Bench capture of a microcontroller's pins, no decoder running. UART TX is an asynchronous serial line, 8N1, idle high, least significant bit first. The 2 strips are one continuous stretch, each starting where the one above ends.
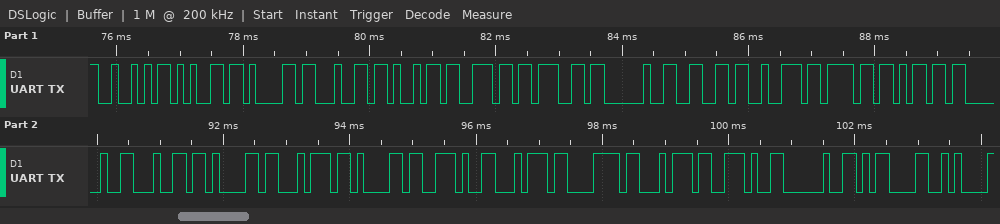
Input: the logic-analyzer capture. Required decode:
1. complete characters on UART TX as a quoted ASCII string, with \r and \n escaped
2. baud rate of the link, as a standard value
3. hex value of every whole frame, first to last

"Reading from data.txt. \r\n"
9600 baud
52 65 61 64 69 6E 67 20 66 72 6F 6D 20 64 61 74 61 2E 74 78 74 2E 20 0D 0A
